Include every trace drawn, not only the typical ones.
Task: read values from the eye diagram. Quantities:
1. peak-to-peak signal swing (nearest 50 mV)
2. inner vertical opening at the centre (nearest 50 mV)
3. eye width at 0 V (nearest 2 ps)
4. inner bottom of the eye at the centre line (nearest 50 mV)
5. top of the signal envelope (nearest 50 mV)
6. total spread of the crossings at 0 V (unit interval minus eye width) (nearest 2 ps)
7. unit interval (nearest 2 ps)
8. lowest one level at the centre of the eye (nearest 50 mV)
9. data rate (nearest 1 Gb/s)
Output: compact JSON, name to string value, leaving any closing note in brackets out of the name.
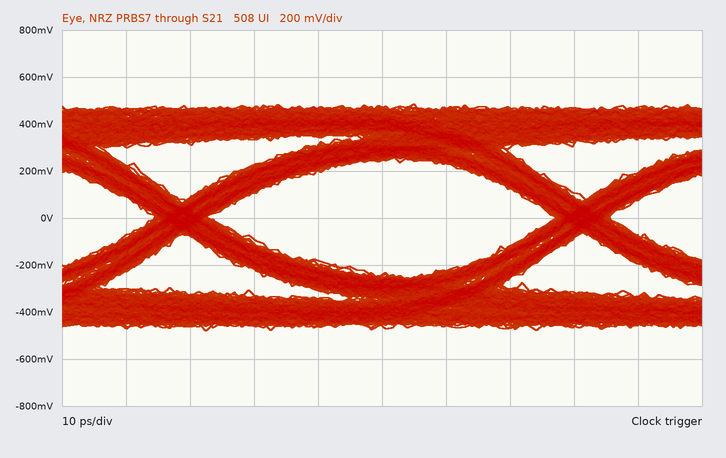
{"peak-to-peak signal swing": "950 mV", "inner vertical opening at the centre": "500 mV", "eye width at 0 V": "54 ps", "inner bottom of the eye at the centre line": "-250 mV", "top of the signal envelope": "500 mV", "total spread of the crossings at 0 V (unit interval minus eye width)": "8 ps", "unit interval": "62 ps", "lowest one level at the centre of the eye": "250 mV", "data rate": "16 Gb/s"}
